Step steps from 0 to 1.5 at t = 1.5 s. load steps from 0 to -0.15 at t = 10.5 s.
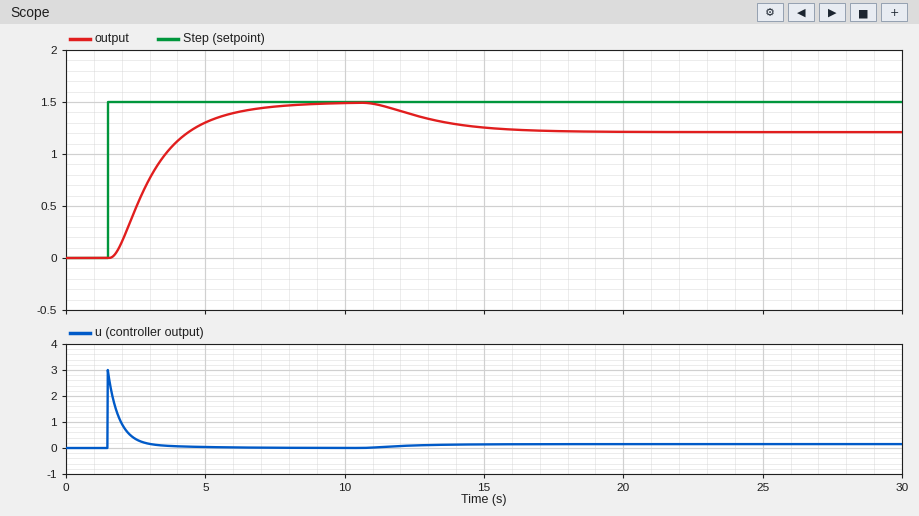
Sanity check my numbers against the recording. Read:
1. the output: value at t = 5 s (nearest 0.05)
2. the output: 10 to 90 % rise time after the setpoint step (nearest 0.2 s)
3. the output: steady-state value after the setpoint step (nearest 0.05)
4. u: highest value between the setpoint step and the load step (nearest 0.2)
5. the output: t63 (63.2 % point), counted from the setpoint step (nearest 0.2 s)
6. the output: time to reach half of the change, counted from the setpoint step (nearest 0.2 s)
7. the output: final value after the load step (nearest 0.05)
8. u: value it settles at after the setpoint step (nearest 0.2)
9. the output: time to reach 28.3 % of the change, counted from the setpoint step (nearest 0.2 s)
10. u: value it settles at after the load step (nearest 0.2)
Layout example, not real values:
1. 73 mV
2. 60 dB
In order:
1. 1.30
2. 3.4 s
3. 1.50
4. 3.0
5. 2.0 s
6. 1.4 s
7. 1.20
8. 0.0
9. 1.0 s
10. 0.2
